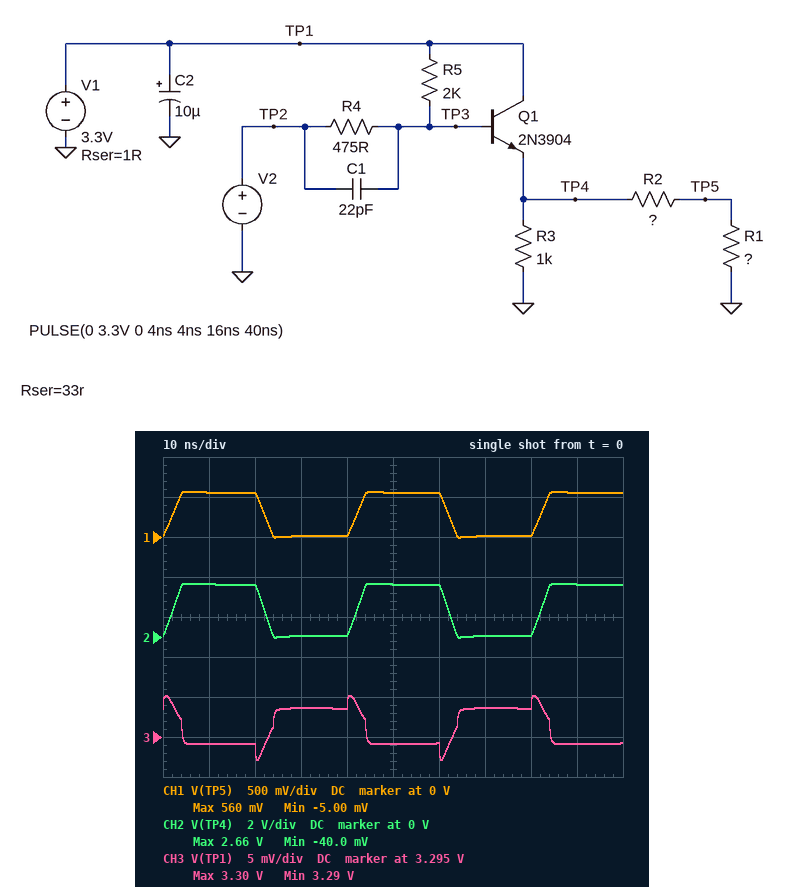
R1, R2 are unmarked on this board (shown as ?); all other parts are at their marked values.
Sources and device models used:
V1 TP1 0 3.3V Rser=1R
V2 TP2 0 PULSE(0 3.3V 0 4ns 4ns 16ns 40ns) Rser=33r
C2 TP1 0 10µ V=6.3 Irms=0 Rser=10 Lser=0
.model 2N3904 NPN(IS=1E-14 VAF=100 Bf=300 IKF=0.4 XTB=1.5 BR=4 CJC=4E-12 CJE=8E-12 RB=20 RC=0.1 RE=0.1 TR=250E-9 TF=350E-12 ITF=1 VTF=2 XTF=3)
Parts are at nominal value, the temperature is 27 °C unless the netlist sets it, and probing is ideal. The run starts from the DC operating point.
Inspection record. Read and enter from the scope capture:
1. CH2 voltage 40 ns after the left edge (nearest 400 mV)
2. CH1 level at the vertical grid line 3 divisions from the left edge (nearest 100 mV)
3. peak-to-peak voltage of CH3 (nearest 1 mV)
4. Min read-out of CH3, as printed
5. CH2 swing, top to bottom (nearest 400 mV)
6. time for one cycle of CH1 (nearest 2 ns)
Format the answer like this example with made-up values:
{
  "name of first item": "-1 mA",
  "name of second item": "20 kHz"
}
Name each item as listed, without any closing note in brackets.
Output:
{
  "CH2 voltage 40 ns after the left edge": "0 V",
  "CH1 level at the vertical grid line 3 divisions from the left edge": "0 V",
  "peak-to-peak voltage of CH3": "8 mV",
  "Min read-out of CH3, as printed": "3.29 V",
  "CH2 swing, top to bottom": "2.8 V",
  "time for one cycle of CH1": "40 ns"
}
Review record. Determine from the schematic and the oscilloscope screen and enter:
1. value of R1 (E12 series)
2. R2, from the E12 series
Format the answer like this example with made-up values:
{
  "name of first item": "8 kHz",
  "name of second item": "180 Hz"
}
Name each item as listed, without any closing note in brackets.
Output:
{
  "value of R1": "150 Ω",
  "R2, from the E12 series": "560 Ω"
}
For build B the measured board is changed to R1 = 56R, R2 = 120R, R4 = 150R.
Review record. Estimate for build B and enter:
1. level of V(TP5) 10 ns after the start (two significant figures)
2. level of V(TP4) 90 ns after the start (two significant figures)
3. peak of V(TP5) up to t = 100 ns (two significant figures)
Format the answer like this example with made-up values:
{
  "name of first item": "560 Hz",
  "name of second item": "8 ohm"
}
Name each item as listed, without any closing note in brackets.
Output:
{
  "level of V(TP5) 10 ns after the start": "790 mV",
  "level of V(TP4) 90 ns after the start": "2.5 V",
  "peak of V(TP5) up to t = 100 ns": "810 mV"
}
